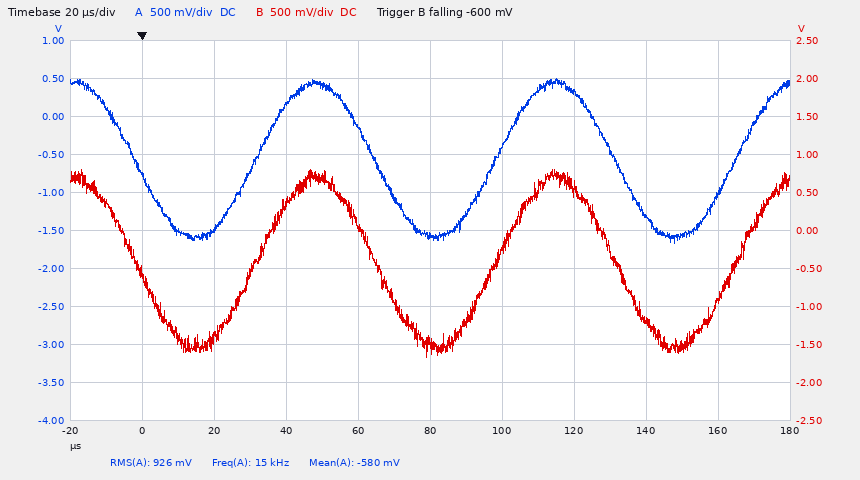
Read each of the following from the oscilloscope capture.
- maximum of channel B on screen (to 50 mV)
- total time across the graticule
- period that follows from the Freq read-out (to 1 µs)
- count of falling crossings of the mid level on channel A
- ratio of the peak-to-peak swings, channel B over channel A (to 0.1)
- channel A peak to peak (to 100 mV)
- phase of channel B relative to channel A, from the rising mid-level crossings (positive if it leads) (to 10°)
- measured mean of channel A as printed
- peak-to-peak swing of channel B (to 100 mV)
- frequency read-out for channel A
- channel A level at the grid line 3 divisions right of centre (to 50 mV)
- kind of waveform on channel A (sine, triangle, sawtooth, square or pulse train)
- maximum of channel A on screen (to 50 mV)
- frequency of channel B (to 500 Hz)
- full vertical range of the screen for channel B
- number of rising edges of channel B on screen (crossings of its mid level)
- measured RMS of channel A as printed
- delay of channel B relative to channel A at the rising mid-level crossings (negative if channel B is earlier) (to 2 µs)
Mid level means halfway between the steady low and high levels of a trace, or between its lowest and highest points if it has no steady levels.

800 mV
200 µs
67 µs
3
1.1
2.20 V
0°
-580 mV
2.50 V
15 kHz
-1.30 V
sine
500 mV
15.0 kHz
5 V
3
926 mV
0 µs
